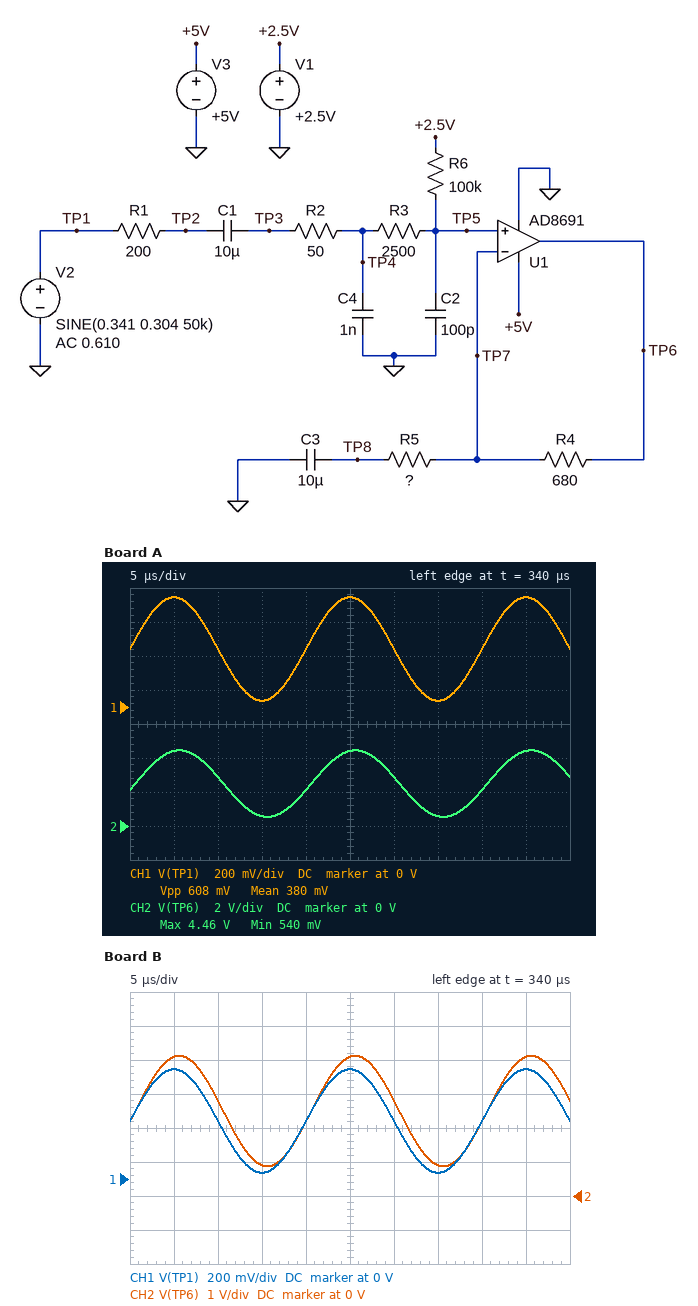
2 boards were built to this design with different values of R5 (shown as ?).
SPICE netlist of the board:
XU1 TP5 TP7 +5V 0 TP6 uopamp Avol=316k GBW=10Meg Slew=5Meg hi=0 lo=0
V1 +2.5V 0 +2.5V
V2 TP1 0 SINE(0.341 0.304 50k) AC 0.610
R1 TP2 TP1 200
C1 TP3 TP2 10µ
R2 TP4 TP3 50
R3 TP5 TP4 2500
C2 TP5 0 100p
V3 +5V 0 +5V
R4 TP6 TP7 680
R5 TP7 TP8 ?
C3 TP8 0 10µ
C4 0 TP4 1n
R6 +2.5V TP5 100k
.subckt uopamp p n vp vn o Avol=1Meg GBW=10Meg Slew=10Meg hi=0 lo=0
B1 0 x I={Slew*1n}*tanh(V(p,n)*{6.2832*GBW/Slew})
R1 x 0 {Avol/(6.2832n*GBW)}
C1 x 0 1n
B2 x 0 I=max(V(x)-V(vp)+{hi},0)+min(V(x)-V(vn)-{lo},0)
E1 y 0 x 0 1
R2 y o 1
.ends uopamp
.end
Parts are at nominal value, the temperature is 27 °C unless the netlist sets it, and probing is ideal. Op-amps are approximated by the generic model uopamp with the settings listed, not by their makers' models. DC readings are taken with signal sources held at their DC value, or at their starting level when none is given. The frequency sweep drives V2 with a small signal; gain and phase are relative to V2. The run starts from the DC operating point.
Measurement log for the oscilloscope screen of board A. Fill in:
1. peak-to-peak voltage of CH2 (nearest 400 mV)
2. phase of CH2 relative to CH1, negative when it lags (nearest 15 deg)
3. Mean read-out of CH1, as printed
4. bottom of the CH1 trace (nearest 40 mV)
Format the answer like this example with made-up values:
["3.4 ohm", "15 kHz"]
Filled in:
["4.0 V", "-15 deg", "380 mV", "40 mV"]
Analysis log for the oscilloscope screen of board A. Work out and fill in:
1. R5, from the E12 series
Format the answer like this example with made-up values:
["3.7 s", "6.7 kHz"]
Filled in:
["120 Ω"]
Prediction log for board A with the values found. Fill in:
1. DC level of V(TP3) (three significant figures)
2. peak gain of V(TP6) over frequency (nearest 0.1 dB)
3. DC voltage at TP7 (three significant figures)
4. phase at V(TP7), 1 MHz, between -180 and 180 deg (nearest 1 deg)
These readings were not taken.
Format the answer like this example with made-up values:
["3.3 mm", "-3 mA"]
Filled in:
["2.50 V", "16.2 dB", "2.50 V", "-147 deg"]
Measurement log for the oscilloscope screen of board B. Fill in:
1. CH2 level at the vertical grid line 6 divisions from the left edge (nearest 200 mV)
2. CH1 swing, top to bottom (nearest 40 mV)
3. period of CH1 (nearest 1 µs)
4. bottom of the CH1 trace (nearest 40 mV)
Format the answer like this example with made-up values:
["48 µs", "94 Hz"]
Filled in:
["2.8 V", "600 mV", "20 µs", "40 mV"]
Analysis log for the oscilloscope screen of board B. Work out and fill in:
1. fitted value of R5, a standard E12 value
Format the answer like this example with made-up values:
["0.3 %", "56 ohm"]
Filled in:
["150 Ω"]
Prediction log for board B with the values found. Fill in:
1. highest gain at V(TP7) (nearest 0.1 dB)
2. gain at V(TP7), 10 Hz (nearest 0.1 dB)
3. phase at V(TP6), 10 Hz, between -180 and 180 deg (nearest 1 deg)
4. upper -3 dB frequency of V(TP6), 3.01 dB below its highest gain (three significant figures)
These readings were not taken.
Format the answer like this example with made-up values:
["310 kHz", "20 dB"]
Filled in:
["-0.2 dB", "-0.2 dB", "23 deg", "374 kHz"]
